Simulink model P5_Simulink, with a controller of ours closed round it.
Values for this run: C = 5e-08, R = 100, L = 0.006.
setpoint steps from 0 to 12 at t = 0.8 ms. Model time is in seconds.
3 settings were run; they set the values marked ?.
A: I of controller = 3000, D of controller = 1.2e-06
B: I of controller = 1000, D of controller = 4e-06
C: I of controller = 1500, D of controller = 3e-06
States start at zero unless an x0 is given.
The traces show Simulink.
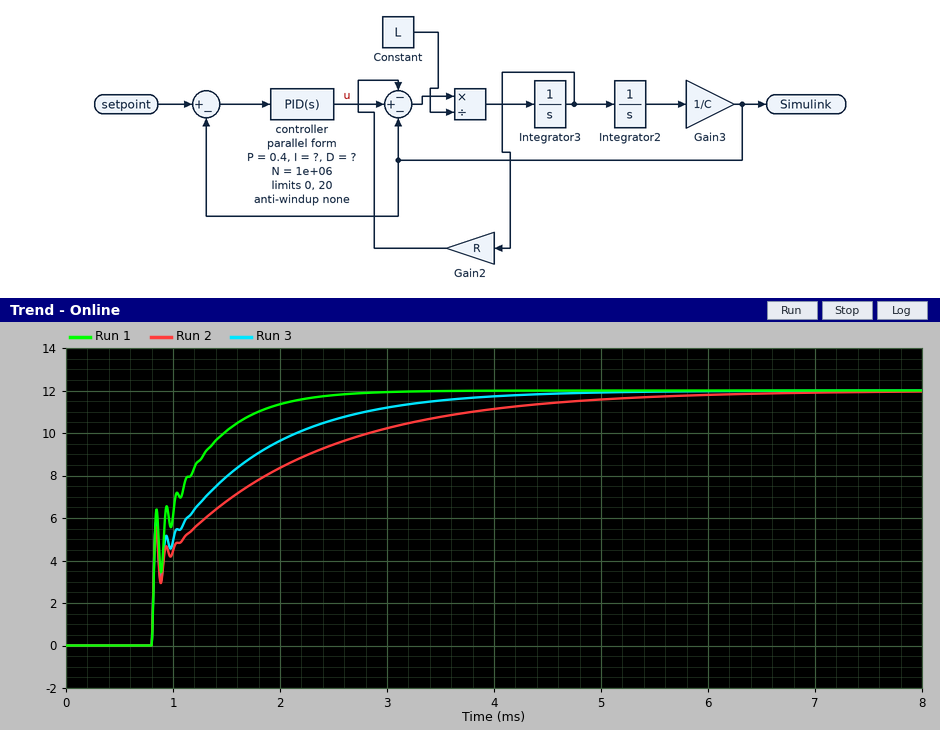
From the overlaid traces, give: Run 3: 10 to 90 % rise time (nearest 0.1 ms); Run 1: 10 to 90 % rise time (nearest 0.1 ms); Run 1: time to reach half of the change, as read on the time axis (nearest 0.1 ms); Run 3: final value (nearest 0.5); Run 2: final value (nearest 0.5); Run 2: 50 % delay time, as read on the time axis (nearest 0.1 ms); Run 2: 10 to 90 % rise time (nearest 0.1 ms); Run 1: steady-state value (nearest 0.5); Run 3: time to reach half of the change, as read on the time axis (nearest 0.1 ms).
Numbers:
1.8 ms
0.9 ms
0.8 ms
12.0
12.0
1.3 ms
2.7 ms
12.0
1.1 ms
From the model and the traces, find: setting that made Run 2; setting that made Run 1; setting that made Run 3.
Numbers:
B
A
C
